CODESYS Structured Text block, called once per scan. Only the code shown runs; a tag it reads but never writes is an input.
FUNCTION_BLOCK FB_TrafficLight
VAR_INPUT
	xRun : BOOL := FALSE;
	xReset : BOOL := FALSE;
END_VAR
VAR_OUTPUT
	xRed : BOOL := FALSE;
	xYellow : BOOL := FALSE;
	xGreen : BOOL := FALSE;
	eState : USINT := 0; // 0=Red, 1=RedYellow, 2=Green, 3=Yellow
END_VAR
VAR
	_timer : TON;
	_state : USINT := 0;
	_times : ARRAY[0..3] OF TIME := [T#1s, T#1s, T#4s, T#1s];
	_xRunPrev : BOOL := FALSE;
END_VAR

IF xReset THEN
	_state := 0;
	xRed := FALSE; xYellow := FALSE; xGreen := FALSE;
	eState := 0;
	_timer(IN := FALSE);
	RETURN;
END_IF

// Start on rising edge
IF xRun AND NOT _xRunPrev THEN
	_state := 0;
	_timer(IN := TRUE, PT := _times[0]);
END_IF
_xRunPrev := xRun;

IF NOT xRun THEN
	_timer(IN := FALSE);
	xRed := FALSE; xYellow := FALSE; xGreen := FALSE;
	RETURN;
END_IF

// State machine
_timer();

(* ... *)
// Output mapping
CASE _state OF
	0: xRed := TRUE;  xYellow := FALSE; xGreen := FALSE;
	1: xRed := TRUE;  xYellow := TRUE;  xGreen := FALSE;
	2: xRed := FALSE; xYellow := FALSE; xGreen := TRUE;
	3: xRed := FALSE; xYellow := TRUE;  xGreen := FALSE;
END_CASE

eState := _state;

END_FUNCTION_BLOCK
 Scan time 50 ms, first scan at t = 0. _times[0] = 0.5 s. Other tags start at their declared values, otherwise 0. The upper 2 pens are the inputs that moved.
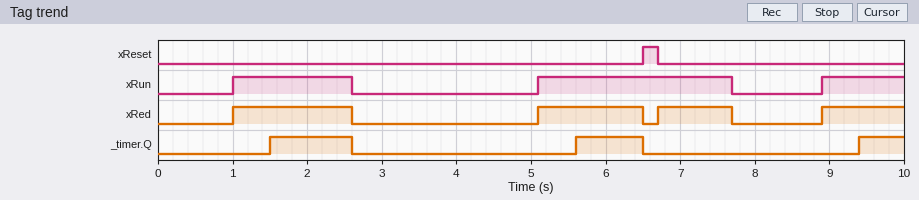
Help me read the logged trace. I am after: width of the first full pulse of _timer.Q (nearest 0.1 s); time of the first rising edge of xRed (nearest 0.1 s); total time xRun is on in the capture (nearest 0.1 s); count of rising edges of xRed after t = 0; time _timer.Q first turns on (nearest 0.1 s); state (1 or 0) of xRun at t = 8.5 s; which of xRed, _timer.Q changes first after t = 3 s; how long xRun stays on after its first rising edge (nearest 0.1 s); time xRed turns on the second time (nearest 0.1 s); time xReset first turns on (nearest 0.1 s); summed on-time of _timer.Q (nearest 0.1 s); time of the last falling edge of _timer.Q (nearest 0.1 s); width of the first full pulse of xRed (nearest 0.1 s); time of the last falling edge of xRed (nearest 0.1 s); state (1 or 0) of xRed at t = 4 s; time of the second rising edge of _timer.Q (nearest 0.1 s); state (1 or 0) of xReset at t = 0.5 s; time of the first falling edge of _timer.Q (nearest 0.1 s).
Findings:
1.1 s
1.0 s
5.3 s
4
1.5 s
0
xRed
1.6 s
5.1 s
6.5 s
2.6 s
6.5 s
1.6 s
7.7 s
0
5.6 s
0
2.6 s
